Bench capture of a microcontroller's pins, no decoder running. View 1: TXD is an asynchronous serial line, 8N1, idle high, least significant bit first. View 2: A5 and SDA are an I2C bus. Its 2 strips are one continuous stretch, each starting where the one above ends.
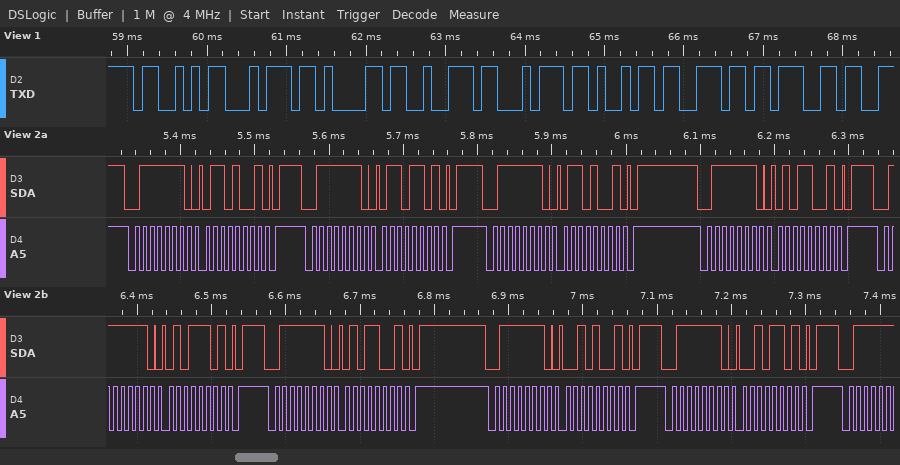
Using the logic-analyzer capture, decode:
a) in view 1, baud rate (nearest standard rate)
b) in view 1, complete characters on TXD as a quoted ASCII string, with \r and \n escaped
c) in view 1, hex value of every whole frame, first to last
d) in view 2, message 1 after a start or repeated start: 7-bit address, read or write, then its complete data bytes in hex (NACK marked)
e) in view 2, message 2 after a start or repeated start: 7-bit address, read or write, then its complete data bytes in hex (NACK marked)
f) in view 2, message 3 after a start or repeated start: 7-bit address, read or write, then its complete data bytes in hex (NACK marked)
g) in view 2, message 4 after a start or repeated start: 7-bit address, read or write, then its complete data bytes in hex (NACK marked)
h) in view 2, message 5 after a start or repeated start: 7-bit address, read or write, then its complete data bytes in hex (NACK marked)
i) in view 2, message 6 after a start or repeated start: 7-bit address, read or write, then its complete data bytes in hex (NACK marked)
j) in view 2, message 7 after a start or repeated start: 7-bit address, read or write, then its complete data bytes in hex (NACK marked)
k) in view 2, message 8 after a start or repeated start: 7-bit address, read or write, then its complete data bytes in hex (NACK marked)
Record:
9600 baud
"Starting"
53 74 61 72 74 69 6E 67
0x3F write: 69
0x3F write: 6D
0x3F write: 69
0x3F write: 59
0x3F write: 5D
0x3F write: 59
0x3F write: 29
0x3F write: 2D
